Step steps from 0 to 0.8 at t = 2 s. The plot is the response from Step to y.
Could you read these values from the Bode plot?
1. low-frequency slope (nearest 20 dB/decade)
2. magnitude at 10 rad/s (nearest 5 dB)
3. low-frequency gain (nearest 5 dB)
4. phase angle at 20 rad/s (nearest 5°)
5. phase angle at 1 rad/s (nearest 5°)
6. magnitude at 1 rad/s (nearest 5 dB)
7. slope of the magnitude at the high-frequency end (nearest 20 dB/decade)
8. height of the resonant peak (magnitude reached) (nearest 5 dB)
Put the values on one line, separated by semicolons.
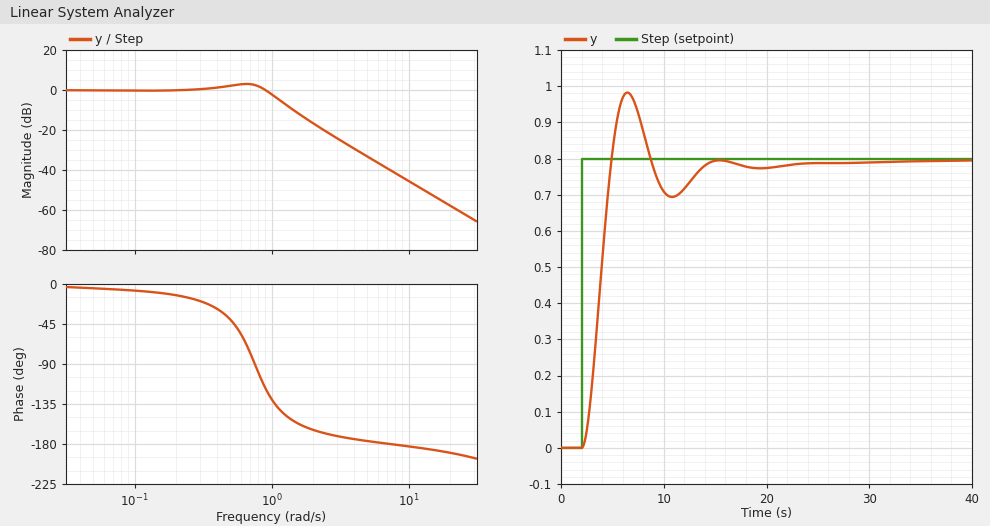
0 dB/decade; -45 dB; 0 dB; -190°; -130°; 0 dB; -40 dB/decade; 5 dB
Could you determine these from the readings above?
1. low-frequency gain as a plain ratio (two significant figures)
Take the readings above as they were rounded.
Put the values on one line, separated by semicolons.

1.0
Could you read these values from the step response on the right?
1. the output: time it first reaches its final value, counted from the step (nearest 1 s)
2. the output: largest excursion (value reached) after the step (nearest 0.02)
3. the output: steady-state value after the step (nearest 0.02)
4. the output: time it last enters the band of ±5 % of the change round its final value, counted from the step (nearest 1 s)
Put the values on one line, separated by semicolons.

3 s; 0.98; 0.80; 11 s
